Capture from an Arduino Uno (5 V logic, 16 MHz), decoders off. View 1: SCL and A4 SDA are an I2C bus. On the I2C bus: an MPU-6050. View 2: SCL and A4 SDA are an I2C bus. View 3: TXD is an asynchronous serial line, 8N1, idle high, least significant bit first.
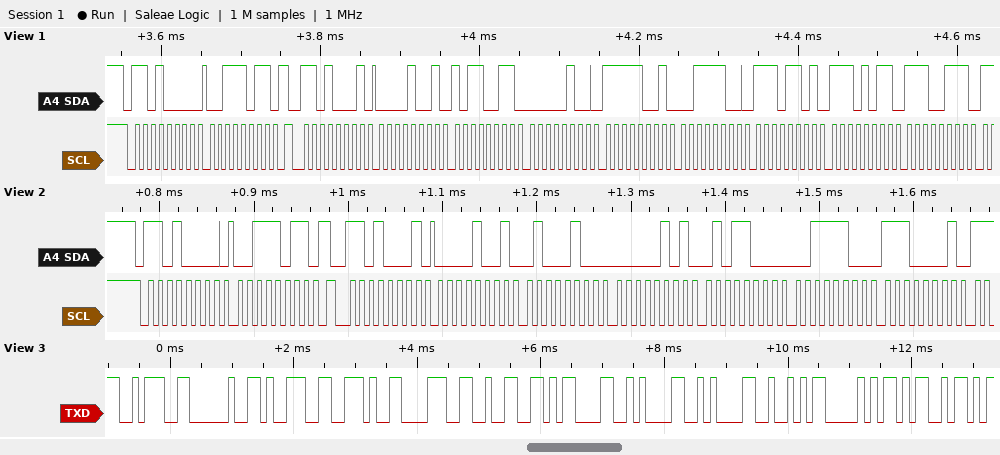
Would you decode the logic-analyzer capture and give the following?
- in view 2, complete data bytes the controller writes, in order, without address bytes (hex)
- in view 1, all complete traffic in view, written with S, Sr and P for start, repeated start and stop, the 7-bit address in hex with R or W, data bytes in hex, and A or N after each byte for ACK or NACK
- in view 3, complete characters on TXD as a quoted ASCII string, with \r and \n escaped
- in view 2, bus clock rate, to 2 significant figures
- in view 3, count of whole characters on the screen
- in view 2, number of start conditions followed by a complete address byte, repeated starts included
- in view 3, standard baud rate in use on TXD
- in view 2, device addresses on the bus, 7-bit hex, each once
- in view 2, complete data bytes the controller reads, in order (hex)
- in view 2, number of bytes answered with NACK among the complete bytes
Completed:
3B
S 68W A 3B A Sr 68R A 09 A B3 A 04 A F9 A 3C A ED A EB A E7 A
": 9.82\r\n\nRPM"
100 kHz
12
2
9600 baud
0x68
09 44 05 58 3C E1
0
